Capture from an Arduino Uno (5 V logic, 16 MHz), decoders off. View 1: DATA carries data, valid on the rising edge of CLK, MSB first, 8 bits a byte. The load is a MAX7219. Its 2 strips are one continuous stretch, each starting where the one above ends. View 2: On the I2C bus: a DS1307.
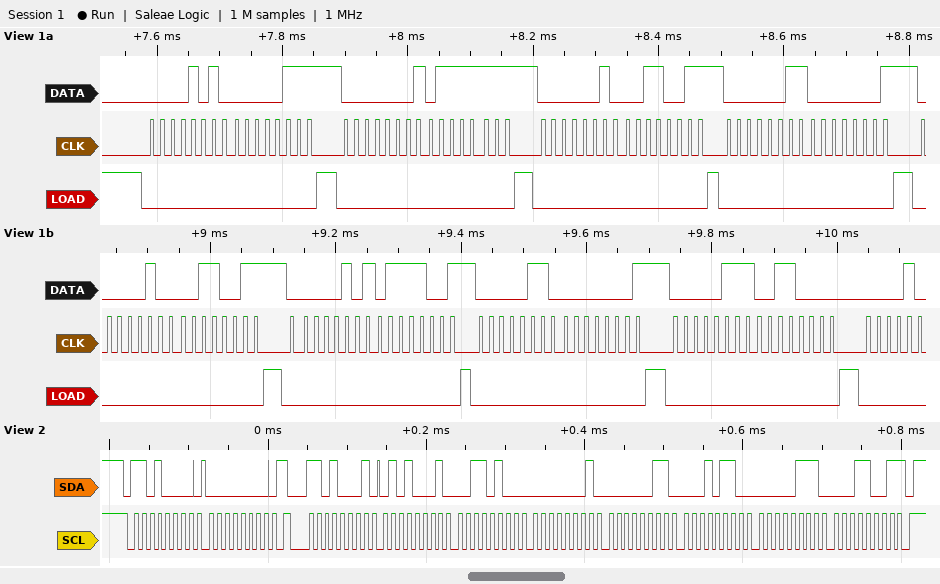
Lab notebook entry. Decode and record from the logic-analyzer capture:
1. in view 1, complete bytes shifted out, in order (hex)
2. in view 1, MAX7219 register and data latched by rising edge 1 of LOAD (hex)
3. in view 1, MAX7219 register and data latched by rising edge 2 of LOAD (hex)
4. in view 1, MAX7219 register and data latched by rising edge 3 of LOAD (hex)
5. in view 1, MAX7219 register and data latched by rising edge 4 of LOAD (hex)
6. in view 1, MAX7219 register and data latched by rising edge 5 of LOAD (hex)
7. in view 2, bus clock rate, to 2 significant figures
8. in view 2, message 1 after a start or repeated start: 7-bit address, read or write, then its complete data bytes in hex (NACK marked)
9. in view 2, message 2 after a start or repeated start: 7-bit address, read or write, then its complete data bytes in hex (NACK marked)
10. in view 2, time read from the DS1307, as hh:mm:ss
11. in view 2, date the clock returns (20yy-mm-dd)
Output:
0A 07 01 7F 02 33 03 01 04 33 05 79 06 01 07 30
register 0xA, data 0x07
register 0x1, data 0x7F
register 0x2, data 0x33
register 0x3, data 0x01
register 0x4, data 0x33
100 kHz
0x68 write: 00
0x68 read: 51 34 01 03 16 07 19 NACK
01:34:51
2019-07-16
